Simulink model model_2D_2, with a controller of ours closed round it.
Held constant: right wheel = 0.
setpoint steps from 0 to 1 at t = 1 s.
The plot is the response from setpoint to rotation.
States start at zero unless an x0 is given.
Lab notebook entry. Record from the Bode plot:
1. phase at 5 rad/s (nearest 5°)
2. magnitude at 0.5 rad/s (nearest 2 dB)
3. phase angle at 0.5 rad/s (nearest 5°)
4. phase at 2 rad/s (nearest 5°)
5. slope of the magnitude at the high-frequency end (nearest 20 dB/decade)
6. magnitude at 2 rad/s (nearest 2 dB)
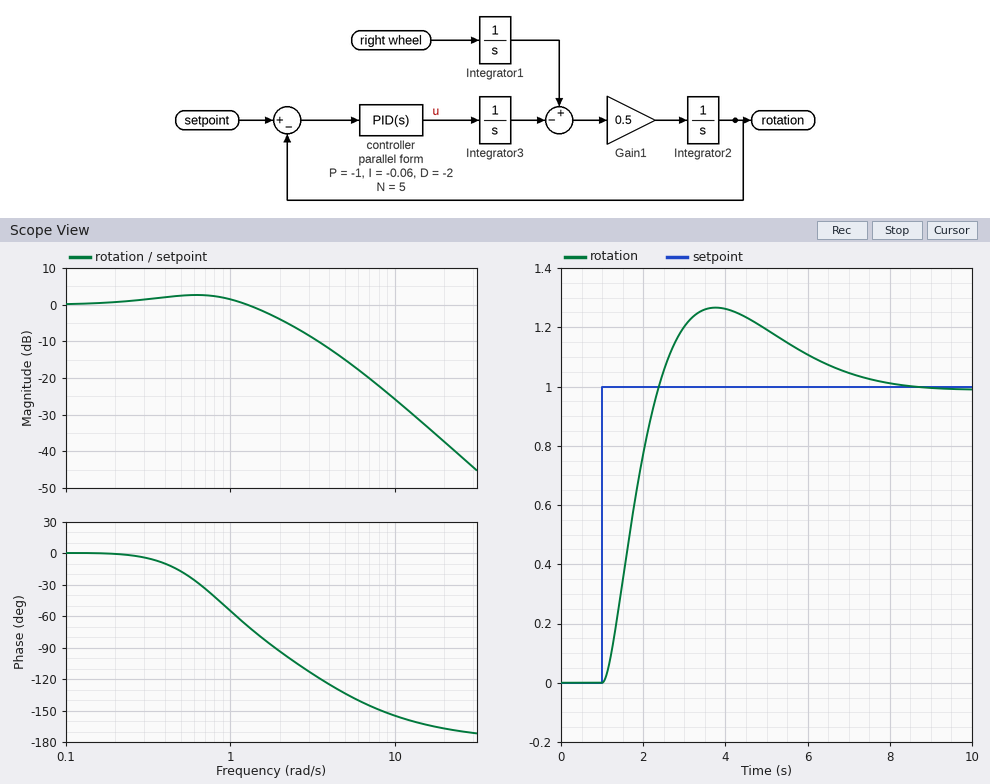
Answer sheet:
-135°
2 dB
-15°
-95°
-40 dB/decade
-4 dB
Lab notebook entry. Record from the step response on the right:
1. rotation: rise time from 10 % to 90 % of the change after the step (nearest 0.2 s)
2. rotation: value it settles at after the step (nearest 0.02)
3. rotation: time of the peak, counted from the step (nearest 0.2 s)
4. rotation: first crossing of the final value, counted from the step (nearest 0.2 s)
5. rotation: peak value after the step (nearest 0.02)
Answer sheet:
1.0 s
1.00
2.8 s
1.4 s
1.26
